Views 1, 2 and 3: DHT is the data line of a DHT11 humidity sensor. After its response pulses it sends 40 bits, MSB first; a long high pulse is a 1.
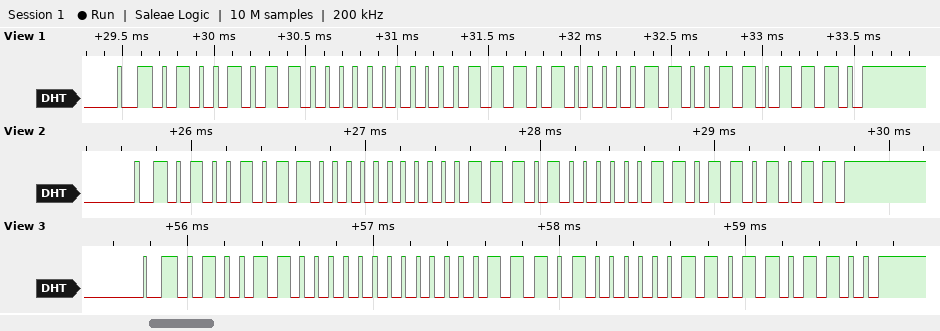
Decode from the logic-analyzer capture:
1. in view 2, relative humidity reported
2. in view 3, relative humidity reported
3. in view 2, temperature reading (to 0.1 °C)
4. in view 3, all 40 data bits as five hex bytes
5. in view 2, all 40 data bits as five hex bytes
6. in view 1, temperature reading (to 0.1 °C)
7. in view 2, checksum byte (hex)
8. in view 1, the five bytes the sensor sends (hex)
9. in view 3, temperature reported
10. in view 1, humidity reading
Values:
75 %
76 %
29.3 °C
4C 00 1D 03 6C
4B 00 1D 03 6B
29.6 °C
0x6B
4B 00 1D 06 6E
29.3 °C
75 %
